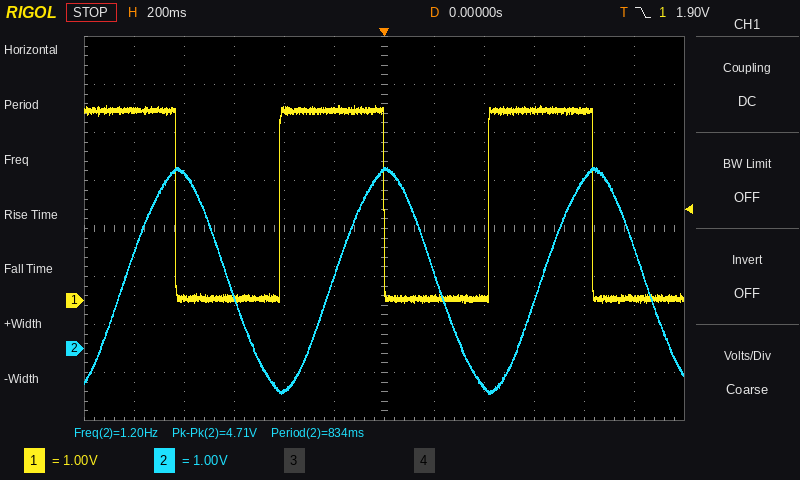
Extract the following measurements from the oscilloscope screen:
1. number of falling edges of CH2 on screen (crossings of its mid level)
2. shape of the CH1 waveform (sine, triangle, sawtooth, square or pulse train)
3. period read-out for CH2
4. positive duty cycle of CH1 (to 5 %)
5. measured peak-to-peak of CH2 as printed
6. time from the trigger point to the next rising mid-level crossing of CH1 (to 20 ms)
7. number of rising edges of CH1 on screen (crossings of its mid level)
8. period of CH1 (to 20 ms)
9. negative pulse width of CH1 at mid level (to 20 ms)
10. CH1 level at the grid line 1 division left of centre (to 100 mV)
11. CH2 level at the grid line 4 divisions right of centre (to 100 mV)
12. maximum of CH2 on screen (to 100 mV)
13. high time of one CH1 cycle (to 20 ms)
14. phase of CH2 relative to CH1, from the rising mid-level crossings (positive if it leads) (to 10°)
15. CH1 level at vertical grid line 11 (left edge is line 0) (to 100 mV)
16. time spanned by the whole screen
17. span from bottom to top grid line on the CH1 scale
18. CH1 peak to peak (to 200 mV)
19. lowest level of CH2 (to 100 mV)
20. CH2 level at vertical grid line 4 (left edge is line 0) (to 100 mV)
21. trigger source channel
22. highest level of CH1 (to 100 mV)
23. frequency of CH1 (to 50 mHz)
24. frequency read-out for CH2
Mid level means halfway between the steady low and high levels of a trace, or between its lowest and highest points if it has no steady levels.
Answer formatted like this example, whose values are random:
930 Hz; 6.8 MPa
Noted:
3; square; 834 ms; 50 %; 4.71 V; 420 ms; 2; 840 ms; 420 ms; 4.0 V; 3.5 V; 3.8 V; 420 ms; -90°; 0.0 V; 2.4 s; 8 V; 4.2 V; -900 mV; -900 mV; CH1; 4.1 V; 1.20 Hz; 1.20 Hz
